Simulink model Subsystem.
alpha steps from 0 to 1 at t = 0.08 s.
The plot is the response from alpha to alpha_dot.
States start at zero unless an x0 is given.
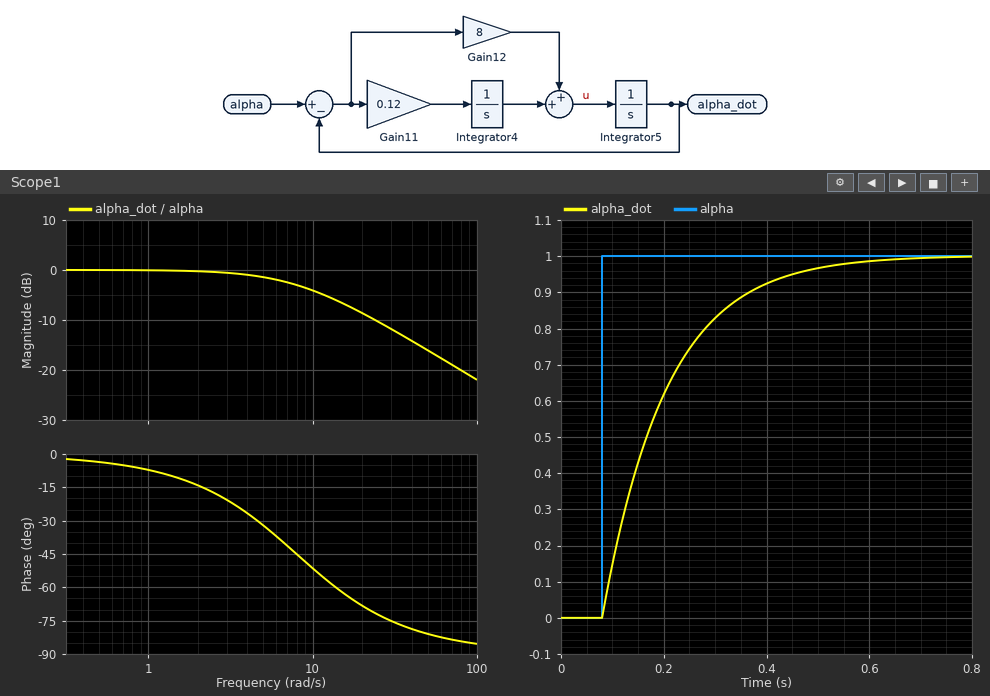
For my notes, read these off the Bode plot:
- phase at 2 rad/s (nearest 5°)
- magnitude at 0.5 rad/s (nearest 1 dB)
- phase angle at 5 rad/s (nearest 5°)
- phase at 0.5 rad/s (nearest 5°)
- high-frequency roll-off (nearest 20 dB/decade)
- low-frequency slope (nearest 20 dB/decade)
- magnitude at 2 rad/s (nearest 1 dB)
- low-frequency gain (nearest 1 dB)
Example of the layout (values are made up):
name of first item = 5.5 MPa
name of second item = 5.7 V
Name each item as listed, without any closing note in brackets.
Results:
phase at 2 rad/s = -15°
magnitude at 0.5 rad/s = 0 dB
phase angle at 5 rad/s = -30°
phase at 0.5 rad/s = -5°
high-frequency roll-off = -20 dB/decade
low-frequency slope = 0 dB/decade
magnitude at 2 rad/s = 0 dB
low-frequency gain = 0 dB
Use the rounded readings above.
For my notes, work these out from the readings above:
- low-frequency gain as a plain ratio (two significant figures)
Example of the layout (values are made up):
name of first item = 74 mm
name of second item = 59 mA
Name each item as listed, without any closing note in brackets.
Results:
low-frequency gain as a plain ratio = 1.0
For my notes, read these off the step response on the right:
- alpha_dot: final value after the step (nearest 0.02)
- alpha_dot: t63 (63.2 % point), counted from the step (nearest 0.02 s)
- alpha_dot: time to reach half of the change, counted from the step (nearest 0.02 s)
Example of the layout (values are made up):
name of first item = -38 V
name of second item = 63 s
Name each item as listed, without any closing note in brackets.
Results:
alpha_dot: final value after the step = 1.00
alpha_dot: t63 (63.2 % point), counted from the step = 0.12 s
alpha_dot: time to reach half of the change, counted from the step = 0.08 s
